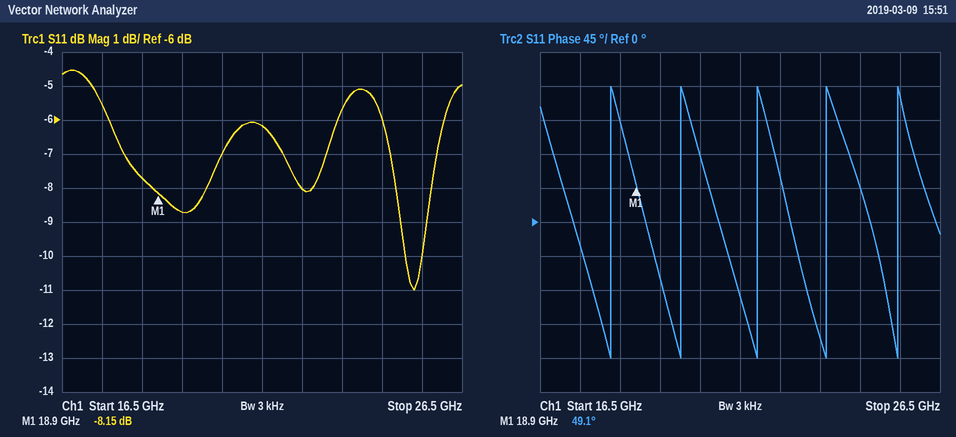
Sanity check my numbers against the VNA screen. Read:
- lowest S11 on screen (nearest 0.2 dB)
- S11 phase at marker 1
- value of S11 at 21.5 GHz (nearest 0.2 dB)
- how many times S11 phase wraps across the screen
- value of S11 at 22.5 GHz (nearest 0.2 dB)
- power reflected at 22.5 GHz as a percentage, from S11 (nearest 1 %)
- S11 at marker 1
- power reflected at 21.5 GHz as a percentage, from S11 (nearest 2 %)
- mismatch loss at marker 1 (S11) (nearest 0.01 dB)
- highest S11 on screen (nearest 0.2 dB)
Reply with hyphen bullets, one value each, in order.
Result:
- -11.0 dB
- 49.1°
- -6.2 dB
- 5
- -8.0 dB
- 16 %
- -8.15 dB
- 24 %
- 0.72 dB
- -4.6 dB
